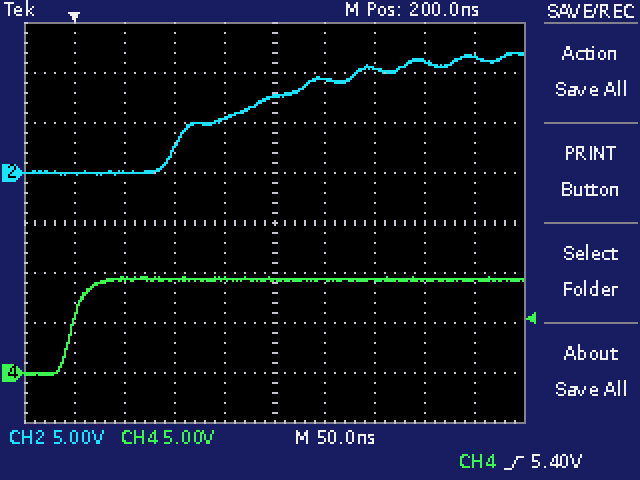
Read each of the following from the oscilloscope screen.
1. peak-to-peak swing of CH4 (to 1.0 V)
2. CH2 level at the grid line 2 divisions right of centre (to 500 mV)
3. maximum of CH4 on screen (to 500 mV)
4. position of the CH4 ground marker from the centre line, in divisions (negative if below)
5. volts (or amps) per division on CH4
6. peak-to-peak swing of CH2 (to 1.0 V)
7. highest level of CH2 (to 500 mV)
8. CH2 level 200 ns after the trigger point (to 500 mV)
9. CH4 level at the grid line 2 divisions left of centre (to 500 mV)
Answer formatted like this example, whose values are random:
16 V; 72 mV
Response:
10.0 V; 10.5 V; 9.5 V; -3.0 div; 5 V; 12.0 V; 12.0 V; 7.5 V; 9.5 V
